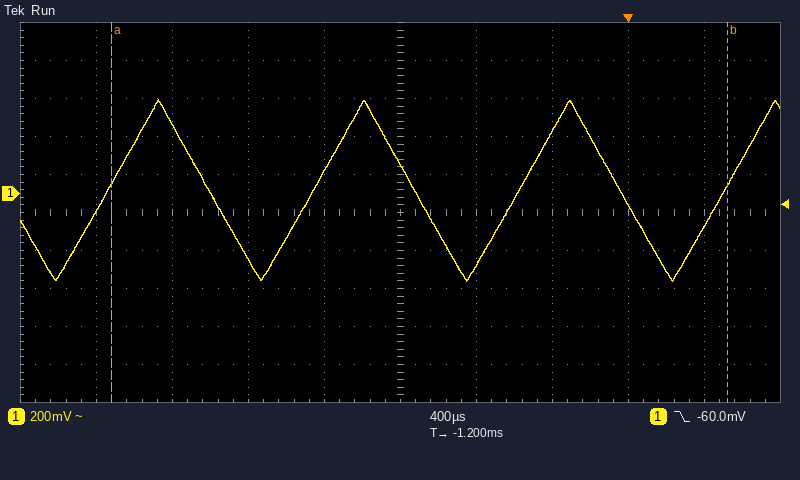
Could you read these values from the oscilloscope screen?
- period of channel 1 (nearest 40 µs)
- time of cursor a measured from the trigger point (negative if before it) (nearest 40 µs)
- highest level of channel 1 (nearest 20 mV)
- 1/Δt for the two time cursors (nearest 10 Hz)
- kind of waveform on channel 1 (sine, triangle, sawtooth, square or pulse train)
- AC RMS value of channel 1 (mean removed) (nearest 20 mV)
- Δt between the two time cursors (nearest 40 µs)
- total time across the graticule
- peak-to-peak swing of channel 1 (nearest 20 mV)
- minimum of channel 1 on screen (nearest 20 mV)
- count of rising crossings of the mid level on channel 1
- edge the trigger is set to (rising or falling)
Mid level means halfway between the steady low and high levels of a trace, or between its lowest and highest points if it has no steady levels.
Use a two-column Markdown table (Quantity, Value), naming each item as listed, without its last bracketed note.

| Quantity | Value |
|---|---|
| period of channel 1 | 1.08 ms |
| time of cursor a measured from the trigger point (negative if before it) | -2.72 ms |
| highest level of channel 1 | 500 mV |
| 1/Δt for the two time cursors | 310 Hz |
| kind of waveform on channel 1 | triangle |
| AC RMS value of channel 1 (mean removed) | 280 mV |
| Δt between the two time cursors | 3.24 ms |
| total time across the graticule | 4 ms |
| peak-to-peak swing of channel 1 | 960 mV |
| minimum of channel 1 on screen | -460 mV |
| count of rising crossings of the mid level on channel 1 | 4 |
| edge the trigger is set to | falling |
